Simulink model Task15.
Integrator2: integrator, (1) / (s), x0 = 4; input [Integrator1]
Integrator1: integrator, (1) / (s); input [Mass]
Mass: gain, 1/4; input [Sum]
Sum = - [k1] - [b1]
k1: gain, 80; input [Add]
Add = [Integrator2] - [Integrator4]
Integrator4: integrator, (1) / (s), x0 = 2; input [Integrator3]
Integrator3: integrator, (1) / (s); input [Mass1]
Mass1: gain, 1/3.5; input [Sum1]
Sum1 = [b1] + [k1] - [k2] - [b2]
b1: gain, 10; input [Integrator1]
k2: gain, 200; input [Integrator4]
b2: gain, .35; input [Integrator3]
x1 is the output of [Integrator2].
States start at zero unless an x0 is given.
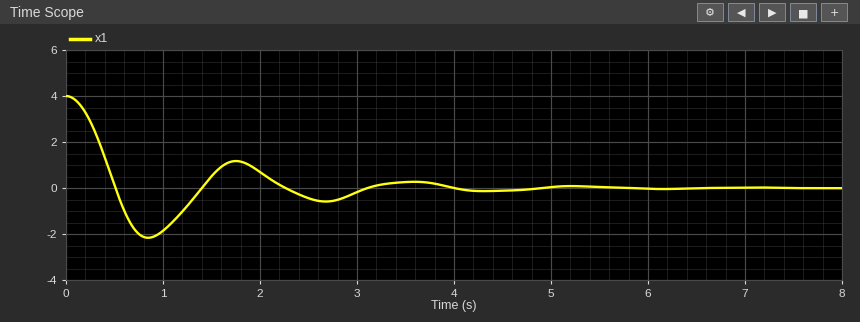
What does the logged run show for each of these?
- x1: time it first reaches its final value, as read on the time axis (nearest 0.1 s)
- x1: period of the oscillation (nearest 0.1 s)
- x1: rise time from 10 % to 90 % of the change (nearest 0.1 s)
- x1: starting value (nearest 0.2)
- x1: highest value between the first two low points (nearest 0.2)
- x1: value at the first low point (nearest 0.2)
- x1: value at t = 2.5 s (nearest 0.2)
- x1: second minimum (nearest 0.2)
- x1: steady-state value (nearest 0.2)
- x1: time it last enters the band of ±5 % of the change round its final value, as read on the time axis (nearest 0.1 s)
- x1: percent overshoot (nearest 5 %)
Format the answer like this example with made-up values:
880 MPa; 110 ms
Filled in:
0.5 s; 1.8 s; 0.3 s; 4.0; 1.2; -2.2; -0.4; -0.6; 0.0; 3.8 s; 55 %
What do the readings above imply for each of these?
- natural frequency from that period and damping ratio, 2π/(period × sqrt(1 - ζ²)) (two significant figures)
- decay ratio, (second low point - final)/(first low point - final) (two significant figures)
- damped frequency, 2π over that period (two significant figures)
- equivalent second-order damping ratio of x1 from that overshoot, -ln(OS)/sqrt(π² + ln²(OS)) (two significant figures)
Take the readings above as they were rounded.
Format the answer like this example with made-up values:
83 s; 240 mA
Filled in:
3.6 rad/s; 0.27; 3.5 rad/s; 0.19
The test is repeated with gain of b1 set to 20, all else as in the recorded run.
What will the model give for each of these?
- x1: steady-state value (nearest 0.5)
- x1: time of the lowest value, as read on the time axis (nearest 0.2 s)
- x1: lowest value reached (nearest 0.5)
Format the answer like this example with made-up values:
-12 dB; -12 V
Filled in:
0.0; 0.8 s; -1.0
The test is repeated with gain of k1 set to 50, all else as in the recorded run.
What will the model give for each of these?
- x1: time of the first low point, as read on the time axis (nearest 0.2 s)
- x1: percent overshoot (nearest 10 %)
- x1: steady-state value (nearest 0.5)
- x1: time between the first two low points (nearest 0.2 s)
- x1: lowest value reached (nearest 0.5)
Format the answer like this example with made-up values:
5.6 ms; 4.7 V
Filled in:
1.0 s; 40 %; 0.0; 2.0 s; -1.5
